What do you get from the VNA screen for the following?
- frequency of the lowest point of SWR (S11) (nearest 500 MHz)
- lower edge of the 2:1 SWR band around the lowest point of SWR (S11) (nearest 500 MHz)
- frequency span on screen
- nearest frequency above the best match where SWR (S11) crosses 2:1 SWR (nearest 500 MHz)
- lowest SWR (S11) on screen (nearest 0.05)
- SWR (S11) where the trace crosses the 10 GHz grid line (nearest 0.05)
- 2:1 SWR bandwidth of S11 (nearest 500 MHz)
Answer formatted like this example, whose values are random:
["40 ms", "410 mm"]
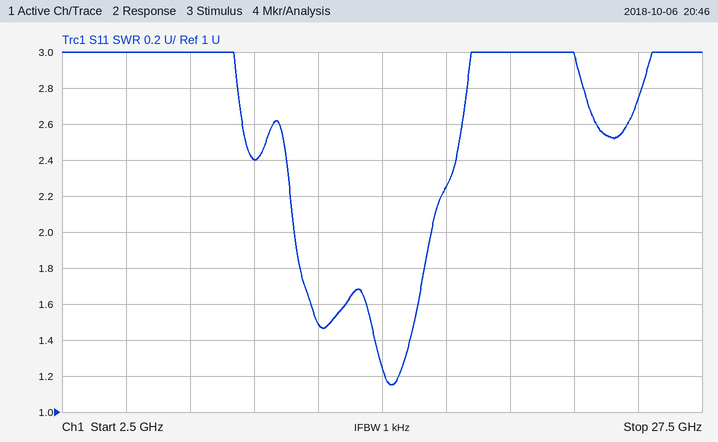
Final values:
["15.5 GHz", "11.5 GHz", "25 GHz", "17.0 GHz", "1.15", "2.40", "5.5 GHz"]
